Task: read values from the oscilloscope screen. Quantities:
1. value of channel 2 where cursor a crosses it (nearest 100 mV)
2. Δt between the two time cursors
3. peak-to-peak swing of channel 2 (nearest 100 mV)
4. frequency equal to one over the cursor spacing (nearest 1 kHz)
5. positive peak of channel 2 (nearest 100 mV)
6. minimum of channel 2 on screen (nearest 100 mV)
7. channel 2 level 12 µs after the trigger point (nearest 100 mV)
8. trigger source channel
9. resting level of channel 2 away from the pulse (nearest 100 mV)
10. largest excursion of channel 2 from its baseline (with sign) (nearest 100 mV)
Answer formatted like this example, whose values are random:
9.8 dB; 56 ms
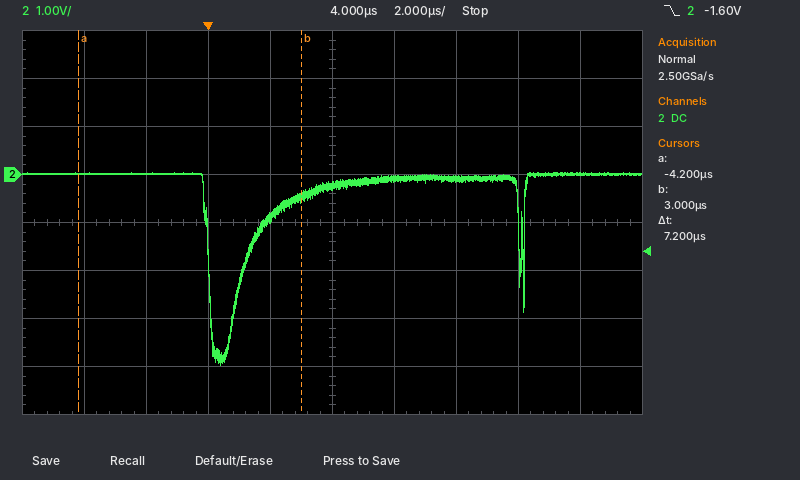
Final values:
0.0 V; 7.2 µs; 4.0 V; 139 kHz; 0.0 V; -4.0 V; 0.0 V; channel 2; 0.0 V; -4.0 V
